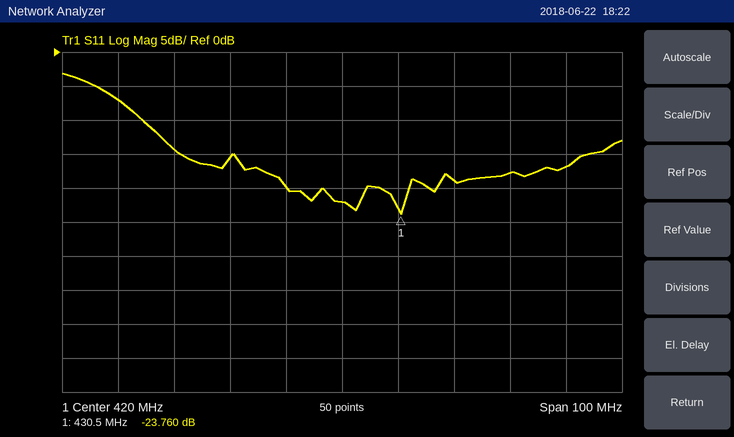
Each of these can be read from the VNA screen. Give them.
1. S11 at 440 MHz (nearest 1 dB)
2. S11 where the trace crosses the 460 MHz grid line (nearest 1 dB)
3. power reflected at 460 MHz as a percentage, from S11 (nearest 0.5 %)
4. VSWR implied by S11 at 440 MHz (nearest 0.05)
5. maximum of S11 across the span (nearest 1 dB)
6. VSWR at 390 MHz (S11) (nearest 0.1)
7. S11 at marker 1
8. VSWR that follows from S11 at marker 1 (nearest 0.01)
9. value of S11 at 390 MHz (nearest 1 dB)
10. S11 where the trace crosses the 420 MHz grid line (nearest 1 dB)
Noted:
-19 dB
-17 dB
2.0 %
1.25
-3 dB
1.5
-23.760 dB
1.14
-14 dB
-22 dB
